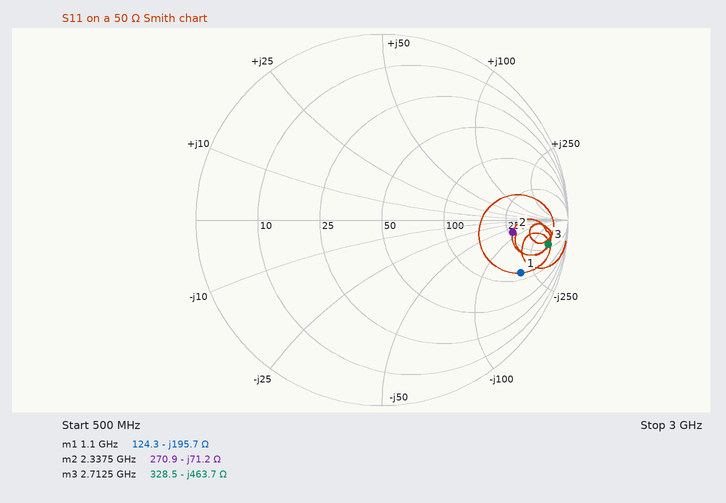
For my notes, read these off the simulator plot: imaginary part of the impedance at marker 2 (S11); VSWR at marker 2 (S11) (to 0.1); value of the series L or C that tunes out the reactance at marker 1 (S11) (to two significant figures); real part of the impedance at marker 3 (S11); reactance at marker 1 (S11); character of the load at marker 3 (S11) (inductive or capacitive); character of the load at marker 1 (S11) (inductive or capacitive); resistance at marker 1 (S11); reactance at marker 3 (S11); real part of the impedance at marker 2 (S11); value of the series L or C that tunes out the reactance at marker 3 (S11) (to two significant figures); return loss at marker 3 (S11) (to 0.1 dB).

-71.2 Ω
5.8
28 nH
328.5 Ω
-195.7 Ω
capacitive
capacitive
124.3 Ω
-463.7 Ω
270.9 Ω
27 nH
0.9 dB
